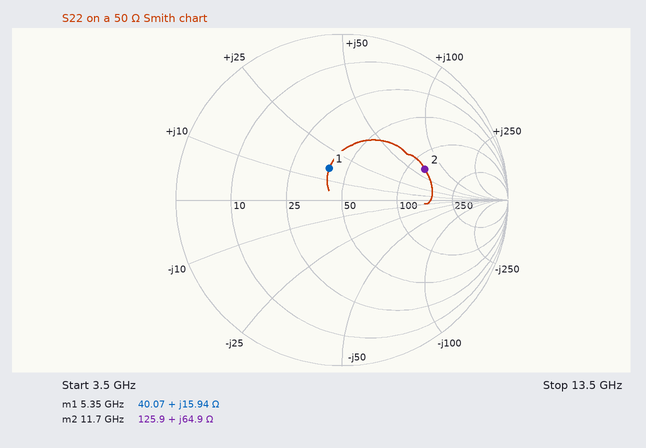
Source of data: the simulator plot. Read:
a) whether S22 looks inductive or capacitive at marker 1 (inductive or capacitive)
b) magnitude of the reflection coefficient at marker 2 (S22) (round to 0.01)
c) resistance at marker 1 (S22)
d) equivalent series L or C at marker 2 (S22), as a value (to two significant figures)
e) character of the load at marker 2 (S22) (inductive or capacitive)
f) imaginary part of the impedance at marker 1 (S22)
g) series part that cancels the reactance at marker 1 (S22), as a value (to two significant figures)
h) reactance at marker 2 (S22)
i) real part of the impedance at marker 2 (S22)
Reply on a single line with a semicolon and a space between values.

inductive; 0.53; 40.07 Ω; 880 pH; inductive; +15.94 Ω; 1.9 pF; +64.9 Ω; 125.9 Ω
